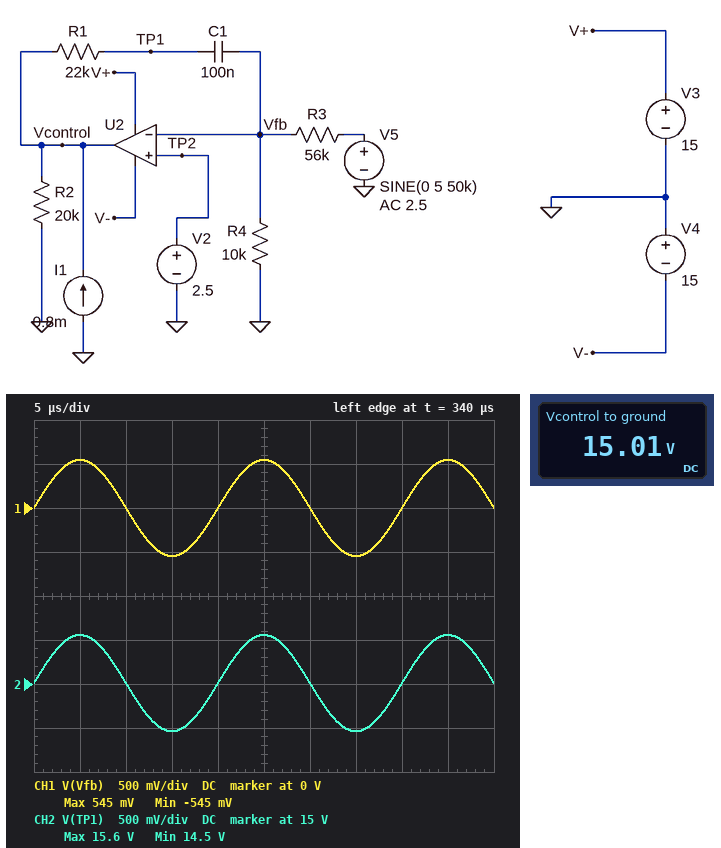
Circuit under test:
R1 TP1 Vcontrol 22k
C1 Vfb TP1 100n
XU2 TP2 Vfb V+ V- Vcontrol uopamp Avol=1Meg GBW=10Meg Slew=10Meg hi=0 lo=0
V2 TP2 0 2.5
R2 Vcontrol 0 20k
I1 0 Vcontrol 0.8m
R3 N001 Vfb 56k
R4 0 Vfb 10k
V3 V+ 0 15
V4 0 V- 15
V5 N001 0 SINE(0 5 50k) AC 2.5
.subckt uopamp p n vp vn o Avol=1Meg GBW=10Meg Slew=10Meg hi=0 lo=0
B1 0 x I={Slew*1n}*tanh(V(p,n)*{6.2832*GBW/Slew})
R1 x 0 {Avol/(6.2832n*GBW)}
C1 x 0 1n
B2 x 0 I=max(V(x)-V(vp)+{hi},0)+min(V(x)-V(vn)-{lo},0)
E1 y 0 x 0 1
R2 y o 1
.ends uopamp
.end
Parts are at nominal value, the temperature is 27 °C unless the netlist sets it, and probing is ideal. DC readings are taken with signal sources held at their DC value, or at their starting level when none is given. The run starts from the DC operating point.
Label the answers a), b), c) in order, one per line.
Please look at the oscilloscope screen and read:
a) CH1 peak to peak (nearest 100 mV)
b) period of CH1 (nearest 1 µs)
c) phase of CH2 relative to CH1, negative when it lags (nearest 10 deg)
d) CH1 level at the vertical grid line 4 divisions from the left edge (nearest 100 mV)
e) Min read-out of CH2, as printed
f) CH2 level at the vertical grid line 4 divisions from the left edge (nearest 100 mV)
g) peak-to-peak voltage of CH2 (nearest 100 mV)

a) 1.1 V
b) 20 µs
c) 0 deg
d) 0 V
e) 14.5 V
f) 15.0 V
g) 1.1 V
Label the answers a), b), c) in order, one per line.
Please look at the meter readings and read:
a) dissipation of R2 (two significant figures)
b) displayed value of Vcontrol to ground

a) 11 mW
b) 15.01 V
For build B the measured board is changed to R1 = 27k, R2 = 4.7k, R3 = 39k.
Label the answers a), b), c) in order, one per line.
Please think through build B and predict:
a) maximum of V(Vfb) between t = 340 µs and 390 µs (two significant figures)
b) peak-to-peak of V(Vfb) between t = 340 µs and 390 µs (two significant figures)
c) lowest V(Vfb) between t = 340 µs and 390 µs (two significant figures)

a) 790 mV
b) 1.6 V
c) -790 mV
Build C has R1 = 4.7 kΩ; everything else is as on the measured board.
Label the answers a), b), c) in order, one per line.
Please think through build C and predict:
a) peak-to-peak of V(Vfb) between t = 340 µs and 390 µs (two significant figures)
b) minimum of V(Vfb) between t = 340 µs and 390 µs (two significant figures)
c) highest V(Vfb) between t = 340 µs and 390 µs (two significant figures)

a) 540 mV
b) -270 mV
c) 270 mV
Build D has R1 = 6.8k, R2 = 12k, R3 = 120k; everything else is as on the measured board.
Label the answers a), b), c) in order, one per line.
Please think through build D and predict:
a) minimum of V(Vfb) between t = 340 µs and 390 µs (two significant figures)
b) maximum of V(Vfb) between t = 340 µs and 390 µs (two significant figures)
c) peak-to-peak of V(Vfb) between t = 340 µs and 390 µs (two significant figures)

a) -160 mV
b) 160 mV
c) 330 mV
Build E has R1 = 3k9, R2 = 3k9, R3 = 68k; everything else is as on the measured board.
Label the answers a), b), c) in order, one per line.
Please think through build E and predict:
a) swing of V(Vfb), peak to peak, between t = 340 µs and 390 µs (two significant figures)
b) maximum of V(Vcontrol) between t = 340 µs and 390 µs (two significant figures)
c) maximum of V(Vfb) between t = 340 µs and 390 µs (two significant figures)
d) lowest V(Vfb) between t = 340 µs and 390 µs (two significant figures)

a) 400 mV
b) 15 V
c) 200 mV
d) -200 mV
